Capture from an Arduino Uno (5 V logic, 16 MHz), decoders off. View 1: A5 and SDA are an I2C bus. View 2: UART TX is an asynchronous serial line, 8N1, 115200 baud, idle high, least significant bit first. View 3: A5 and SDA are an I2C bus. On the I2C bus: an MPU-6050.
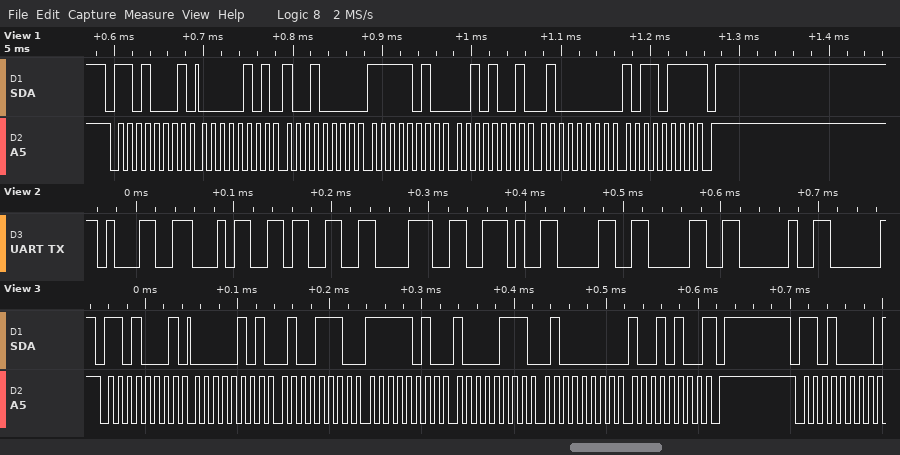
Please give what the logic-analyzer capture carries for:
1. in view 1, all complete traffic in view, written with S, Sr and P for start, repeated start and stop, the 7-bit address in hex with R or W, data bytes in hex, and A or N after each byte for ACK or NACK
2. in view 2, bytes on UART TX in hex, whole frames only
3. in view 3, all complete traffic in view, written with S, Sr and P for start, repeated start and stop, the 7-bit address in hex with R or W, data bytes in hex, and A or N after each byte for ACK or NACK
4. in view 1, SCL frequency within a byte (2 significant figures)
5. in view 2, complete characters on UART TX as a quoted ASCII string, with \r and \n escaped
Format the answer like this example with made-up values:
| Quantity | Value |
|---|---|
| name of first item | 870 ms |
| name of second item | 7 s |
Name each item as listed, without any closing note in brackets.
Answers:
| Quantity | Value |
|---|---|
| in view 1, all complete traffic in view, written with S, Sr and P for start, repeated start and stop, the 7-bit address in hex with R or W, data bytes in hex, and A or N after each byte for ACK or NACK | S 68R A 05 A 90 A FA A 29 A 40 A B7 N P |
| in view 2, bytes on UART TX in hex, whole frames only | 31 34 33 38 2E 30 30 20 |
| in view 3, all complete traffic in view, written with S, Sr and P for start, repeated start and stop, the 7-bit address in hex with R or W, data bytes in hex, and A or N after each byte for ACK or NACK | S 68R A 05 A 4E A FA A 87 A 40 A 94 N P S 68W A |
| in view 1, SCL frequency within a byte | 100 kHz |
| in view 2, complete characters on UART TX as a quoted ASCII string, with \r and \n escaped | "1438.00 " |
